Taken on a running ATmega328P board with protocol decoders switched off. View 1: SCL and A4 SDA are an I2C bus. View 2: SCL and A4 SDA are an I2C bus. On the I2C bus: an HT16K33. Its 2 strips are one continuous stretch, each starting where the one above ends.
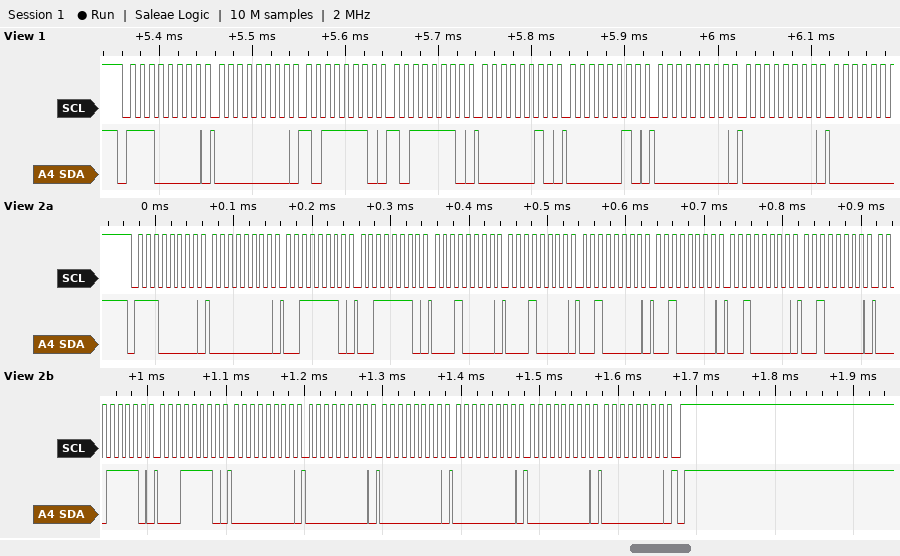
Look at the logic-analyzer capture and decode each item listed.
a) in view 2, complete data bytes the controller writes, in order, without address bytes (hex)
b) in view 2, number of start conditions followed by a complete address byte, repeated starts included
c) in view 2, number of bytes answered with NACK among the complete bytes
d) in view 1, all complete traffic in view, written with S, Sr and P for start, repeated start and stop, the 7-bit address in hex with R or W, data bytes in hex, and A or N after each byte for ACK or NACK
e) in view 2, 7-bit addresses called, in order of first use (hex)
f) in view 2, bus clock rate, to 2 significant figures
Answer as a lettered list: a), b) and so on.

a) 00 3E 3E 10 10 20 20 20 20 1E 1E 00 00 00 00 00 00
b) 1
c) 0
d) S 70W A 00 A BE A BE A 02 A 02 A 00 A 00 A
e) 0x70
f) 100 kHz
